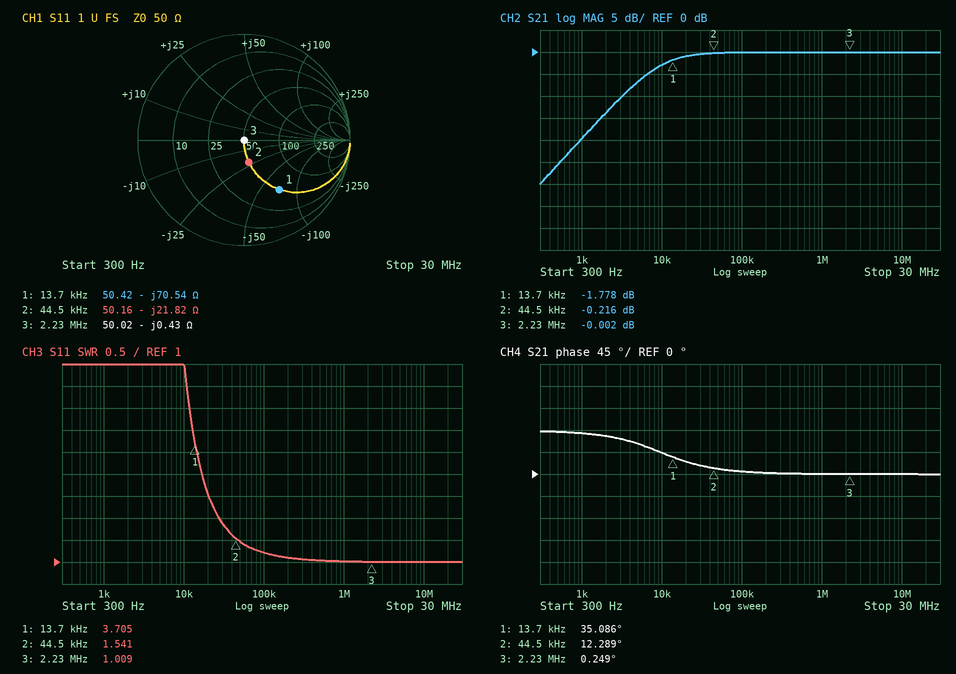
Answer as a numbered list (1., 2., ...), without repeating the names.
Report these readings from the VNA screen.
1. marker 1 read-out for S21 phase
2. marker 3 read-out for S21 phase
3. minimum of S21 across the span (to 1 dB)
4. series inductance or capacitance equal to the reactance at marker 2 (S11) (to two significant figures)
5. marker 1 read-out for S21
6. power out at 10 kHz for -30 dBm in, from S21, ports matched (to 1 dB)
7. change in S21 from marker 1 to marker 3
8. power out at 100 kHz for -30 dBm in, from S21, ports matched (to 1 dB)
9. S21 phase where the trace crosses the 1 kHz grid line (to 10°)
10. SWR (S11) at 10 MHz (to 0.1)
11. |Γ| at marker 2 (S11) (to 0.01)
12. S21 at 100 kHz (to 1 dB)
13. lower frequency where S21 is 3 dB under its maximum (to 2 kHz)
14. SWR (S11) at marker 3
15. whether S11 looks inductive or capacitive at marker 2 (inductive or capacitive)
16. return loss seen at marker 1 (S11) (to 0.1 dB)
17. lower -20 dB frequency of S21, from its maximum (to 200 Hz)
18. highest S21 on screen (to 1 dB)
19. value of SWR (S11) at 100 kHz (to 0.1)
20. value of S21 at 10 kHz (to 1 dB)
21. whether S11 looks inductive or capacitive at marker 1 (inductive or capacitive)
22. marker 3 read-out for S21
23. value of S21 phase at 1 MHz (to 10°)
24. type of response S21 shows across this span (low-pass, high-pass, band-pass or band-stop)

1. 35.086°
2. 0.249°
3. -30 dB
4. 160 nF
5. -1.778 dB
6. -33 dBm
7. 1.776 dB
8. -30 dBm
9. 80°
10. 1.0
11. 0.21
12. 0 dB
13. 10 kHz
14. 1.009
15. capacitive
16. 4.8 dB
17. 1.0 kHz
18. 0 dB
19. 1.2
20. -3 dB
21. capacitive
22. -0.002 dB
23. 0°
24. high-pass
